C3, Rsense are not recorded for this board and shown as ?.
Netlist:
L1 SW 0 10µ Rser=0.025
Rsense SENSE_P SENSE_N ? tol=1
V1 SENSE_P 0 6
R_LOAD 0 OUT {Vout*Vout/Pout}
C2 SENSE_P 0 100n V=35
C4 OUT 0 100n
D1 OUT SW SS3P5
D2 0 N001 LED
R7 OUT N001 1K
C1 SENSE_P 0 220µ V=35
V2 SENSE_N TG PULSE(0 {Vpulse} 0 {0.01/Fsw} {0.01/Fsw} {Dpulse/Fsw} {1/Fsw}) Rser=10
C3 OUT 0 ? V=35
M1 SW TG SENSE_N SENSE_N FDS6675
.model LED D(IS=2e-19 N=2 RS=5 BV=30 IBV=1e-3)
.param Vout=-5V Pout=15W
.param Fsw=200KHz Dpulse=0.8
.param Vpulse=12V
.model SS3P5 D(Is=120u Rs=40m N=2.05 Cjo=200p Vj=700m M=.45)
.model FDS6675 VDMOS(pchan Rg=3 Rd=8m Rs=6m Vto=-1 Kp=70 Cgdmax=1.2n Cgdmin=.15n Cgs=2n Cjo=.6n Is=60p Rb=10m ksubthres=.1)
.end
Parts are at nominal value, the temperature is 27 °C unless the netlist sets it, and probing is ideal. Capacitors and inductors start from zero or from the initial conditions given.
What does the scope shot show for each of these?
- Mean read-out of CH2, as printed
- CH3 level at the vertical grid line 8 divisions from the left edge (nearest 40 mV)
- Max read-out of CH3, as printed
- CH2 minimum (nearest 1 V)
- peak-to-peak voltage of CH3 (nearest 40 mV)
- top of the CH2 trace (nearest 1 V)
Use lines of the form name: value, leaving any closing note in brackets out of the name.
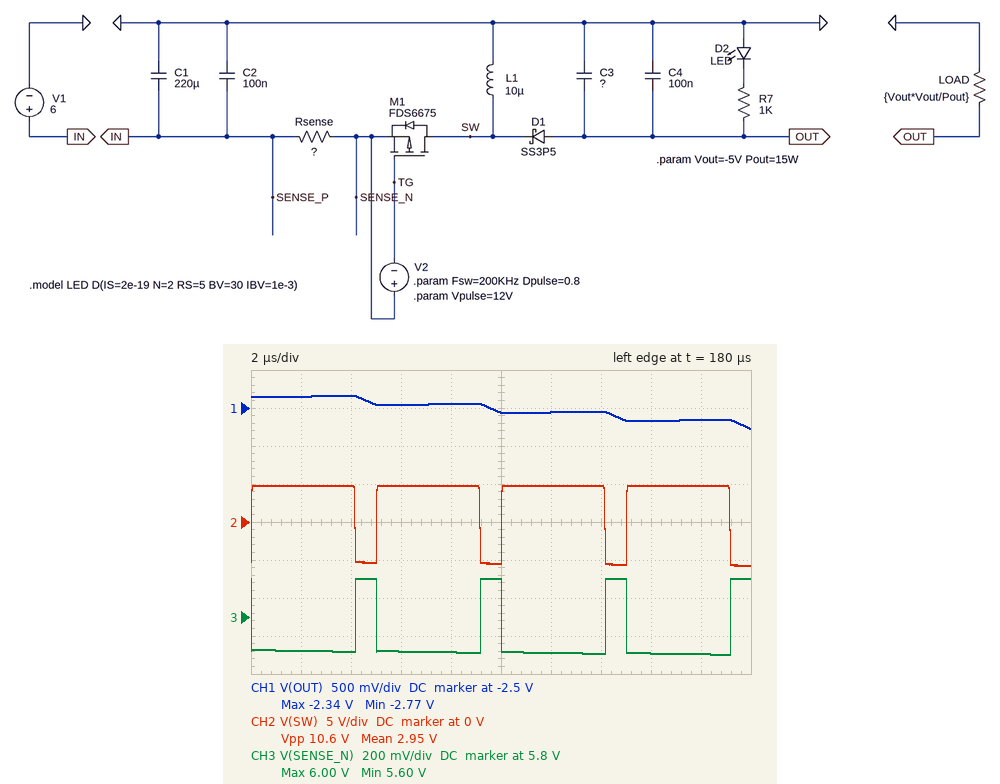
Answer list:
Mean read-out of CH2, as printed: 2.95 V
CH3 level at the vertical grid line 8 divisions from the left edge: 5.60 V
Max read-out of CH3, as printed: 6.00 V
CH2 minimum: -6 V
peak-to-peak voltage of CH3: 400 mV
top of the CH2 trace: 5 V
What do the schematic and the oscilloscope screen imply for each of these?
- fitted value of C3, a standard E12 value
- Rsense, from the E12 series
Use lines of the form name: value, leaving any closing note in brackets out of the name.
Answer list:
fitted value of C3, a standard E12 value: 390 µF
Rsense, from the E12 series: 6.8 mΩ
